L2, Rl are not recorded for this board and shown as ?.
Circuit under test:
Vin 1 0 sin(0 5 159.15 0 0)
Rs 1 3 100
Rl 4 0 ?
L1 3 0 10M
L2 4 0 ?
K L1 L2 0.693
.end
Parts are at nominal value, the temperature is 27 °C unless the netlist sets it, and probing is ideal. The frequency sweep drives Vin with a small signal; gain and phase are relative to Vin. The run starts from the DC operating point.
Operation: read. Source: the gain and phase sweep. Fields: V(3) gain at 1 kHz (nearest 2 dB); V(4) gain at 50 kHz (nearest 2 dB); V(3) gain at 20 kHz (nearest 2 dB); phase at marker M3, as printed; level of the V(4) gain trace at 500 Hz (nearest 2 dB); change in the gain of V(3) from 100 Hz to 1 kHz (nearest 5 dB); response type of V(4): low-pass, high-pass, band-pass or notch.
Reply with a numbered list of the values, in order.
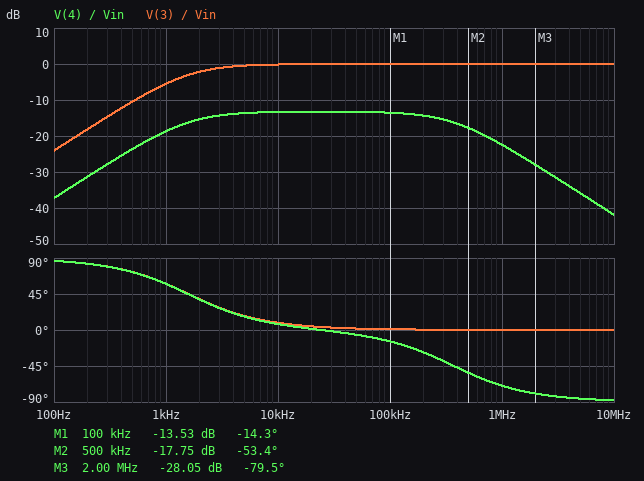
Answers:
1. -6 dB
2. -14 dB
3. 0 dB
4. -79.5 deg
5. -24 dB
6. 20 dB
7. band-pass
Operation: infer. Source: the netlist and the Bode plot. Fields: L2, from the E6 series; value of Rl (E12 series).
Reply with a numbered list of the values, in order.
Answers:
1. 1 mH
2. 1.2 kΩ
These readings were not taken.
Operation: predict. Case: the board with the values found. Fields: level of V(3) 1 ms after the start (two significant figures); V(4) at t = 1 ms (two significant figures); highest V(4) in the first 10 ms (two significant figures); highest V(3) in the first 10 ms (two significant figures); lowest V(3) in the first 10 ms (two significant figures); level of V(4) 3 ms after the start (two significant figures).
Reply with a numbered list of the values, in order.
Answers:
1. 310 mV
2. 68 mV
3. 110 mV
4. 500 mV
5. -500 mV
6. -110 mV
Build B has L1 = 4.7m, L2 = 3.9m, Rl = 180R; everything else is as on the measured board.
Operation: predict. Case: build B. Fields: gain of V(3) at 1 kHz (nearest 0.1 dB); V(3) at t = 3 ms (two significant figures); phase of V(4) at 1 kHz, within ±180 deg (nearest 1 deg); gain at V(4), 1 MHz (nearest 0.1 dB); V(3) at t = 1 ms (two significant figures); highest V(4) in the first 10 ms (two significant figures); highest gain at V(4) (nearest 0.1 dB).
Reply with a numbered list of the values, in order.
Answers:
1. -11.2 dB
2. -230 mV
3. 66 deg
4. -41.0 dB
5. 140 mV
6. 150 mV
7. -7.3 dB
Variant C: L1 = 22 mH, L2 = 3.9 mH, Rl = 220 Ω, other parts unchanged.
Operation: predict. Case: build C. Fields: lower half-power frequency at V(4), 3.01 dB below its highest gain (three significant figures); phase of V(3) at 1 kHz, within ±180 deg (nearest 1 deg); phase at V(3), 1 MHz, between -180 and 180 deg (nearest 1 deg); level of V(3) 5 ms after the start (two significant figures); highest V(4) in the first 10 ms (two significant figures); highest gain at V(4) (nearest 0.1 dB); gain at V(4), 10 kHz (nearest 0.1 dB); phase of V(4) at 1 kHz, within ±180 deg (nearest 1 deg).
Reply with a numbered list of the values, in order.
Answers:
1. 647 Hz
2. 35 deg
3. 0 deg
4. 67 mV
5. 310 mV
6. -11.4 dB
7. -12.2 dB
8. 32 deg
